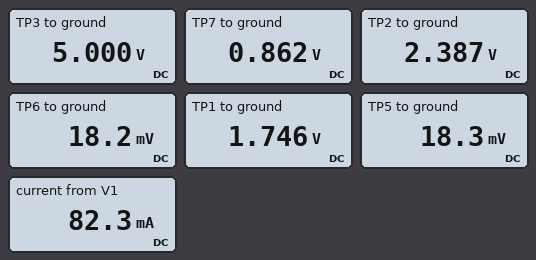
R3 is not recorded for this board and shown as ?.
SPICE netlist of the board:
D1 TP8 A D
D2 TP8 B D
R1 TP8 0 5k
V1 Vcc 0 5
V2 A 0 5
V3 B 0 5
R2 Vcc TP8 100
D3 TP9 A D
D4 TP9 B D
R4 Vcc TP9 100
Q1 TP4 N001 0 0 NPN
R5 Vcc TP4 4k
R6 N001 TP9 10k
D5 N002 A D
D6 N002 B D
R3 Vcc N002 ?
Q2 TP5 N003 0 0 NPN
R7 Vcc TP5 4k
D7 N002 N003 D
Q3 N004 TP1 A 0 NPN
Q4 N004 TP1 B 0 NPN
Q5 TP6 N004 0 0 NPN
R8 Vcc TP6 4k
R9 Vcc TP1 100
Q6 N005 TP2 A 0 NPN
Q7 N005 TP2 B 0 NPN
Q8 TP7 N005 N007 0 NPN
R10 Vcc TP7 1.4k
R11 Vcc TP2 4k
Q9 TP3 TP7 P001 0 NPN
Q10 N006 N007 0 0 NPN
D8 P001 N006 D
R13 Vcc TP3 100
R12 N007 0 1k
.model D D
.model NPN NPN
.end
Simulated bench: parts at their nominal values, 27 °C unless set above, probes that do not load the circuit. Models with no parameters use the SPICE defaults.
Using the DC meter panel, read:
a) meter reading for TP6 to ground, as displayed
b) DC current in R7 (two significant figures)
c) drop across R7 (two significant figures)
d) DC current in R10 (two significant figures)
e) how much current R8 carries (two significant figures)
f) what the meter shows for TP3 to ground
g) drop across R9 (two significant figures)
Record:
18.2 mV
1.2 mA
5.0 V
3.0 mA
1.2 mA
5.000 V
3.3 V
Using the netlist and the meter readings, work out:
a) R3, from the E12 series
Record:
82 Ω
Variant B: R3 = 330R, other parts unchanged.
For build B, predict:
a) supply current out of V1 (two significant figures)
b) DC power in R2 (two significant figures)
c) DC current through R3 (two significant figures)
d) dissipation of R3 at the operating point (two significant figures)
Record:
52 mA
96 µW
10 mA
36 mW
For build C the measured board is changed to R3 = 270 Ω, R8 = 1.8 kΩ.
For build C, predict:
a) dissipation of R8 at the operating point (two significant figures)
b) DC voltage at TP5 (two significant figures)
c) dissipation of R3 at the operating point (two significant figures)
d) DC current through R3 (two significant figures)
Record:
14 mW
19 mV
43 mW
13 mA
